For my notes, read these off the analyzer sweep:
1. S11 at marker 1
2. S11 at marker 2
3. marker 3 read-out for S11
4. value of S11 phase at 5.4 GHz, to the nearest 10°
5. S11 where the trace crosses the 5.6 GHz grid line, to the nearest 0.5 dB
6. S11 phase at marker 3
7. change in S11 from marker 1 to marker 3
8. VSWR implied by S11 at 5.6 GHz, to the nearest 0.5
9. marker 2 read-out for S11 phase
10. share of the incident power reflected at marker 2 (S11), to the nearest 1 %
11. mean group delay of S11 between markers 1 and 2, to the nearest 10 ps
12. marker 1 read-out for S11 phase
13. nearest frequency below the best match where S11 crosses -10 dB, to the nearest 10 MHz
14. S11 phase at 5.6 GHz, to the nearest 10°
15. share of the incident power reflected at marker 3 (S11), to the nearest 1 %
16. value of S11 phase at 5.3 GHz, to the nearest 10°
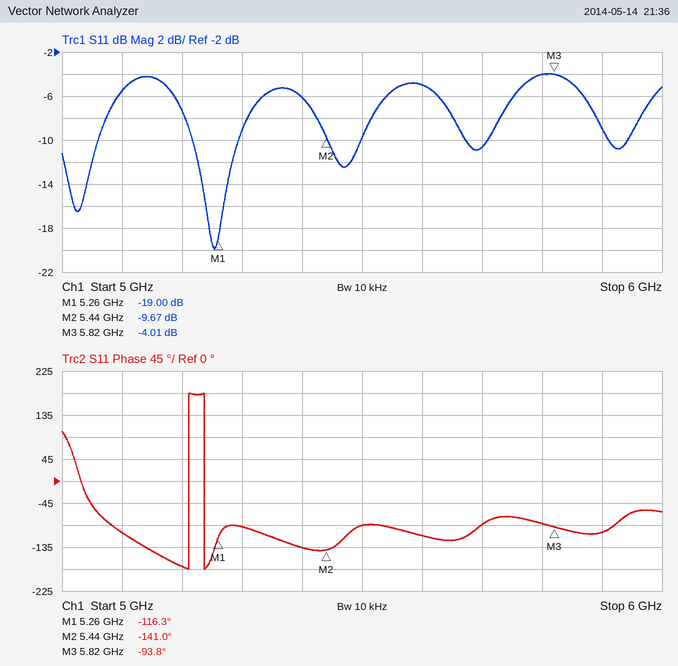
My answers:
-19.00 dB
-9.67 dB
-4.01 dB
-140°
-5.0 dB
-93.8°
14.99 dB
3.5
-141.0°
11 %
380 ps
-116.3°
5.22 GHz
-110°
40 %
-90°
